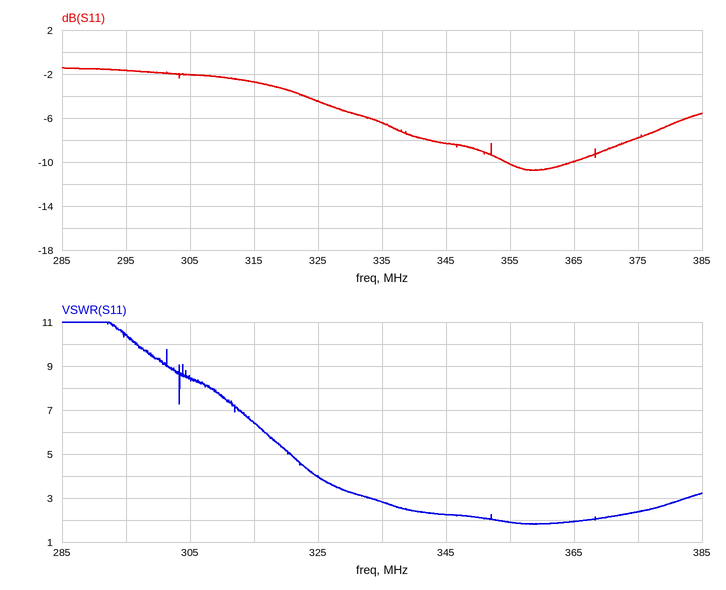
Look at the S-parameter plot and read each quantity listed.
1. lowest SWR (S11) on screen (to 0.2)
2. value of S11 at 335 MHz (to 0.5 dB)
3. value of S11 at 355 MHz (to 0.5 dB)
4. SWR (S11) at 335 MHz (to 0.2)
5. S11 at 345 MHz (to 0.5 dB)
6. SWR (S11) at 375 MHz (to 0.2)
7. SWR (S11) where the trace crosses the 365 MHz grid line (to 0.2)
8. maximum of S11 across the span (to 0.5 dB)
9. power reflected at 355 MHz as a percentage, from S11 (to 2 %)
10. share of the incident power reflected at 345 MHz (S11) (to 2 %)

1.8
-6.5 dB
-10.0 dB
2.8
-8.5 dB
2.4
2.0
-1.5 dB
10 %
14 %
